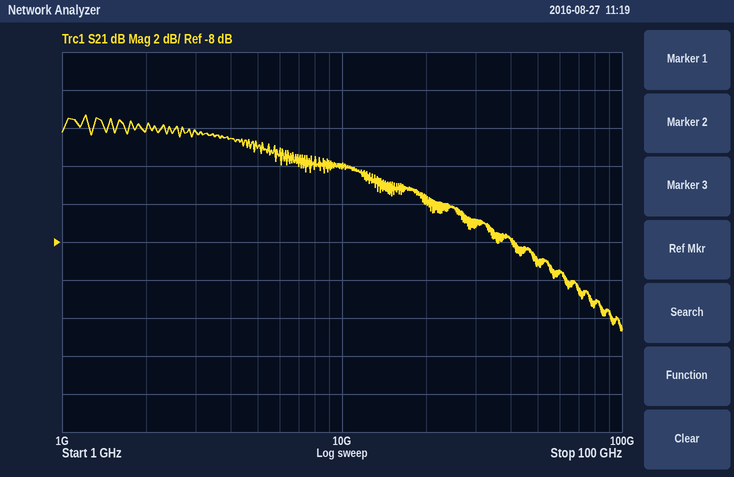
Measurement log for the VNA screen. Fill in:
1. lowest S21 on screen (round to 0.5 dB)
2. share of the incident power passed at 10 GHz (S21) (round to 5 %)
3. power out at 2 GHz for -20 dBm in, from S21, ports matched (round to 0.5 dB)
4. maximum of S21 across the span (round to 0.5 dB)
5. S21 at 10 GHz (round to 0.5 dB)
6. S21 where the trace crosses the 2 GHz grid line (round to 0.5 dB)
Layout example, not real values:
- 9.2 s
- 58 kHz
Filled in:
- -12.5 dB
- 40 %
- -22.0 dBm
- -1.5 dB
- -4.0 dB
- -2.0 dB
